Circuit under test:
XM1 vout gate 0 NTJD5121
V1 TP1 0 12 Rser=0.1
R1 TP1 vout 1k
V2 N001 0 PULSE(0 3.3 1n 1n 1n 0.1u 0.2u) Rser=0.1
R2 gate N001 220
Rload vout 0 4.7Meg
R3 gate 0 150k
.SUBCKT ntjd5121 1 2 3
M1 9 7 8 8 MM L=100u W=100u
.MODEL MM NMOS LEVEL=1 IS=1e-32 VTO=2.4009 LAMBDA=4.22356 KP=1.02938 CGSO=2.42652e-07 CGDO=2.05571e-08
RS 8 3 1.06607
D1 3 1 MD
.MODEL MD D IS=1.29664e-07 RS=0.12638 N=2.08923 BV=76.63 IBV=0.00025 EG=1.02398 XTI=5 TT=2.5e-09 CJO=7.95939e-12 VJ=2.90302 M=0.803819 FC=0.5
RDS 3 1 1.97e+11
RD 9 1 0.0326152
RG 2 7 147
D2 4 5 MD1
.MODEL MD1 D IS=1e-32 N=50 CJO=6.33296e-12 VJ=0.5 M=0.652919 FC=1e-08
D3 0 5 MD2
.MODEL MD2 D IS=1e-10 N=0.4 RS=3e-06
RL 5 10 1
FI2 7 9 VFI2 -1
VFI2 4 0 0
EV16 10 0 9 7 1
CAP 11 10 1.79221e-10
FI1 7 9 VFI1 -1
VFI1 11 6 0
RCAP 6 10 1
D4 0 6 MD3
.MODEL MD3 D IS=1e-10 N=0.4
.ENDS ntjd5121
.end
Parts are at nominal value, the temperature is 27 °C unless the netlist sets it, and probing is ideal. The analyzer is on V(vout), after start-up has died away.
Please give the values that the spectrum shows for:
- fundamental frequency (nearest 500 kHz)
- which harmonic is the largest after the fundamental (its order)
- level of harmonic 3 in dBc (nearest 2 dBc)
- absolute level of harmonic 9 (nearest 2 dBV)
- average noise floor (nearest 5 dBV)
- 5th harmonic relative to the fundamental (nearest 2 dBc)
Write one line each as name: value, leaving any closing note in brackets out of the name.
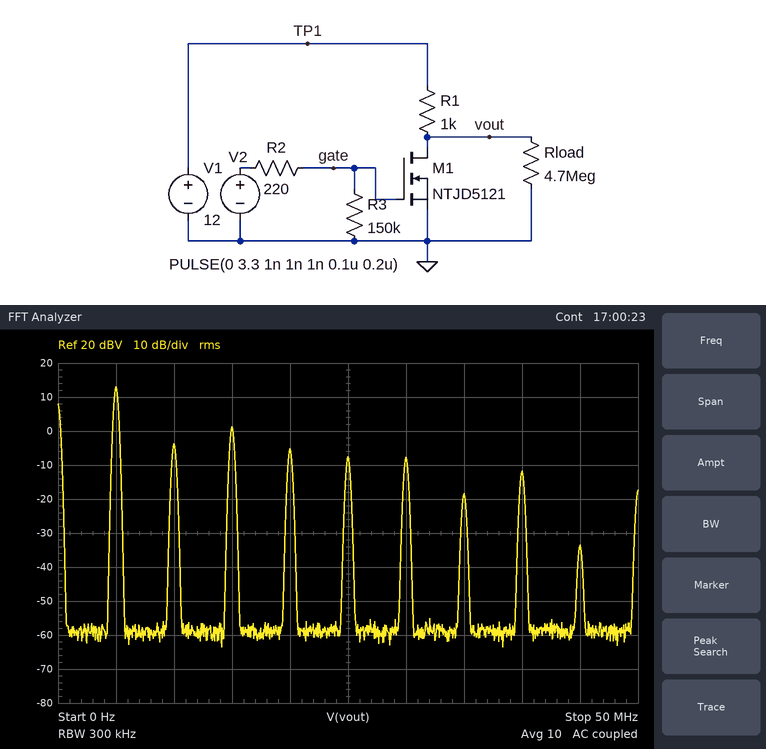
fundamental frequency: 5.0 MHz
which harmonic is the largest after the fundamental: 3
level of harmonic 3 in dBc: -12 dBc
absolute level of harmonic 9: -34 dBV
average noise floor: -60 dBV
5th harmonic relative to the fundamental: -20 dBc
